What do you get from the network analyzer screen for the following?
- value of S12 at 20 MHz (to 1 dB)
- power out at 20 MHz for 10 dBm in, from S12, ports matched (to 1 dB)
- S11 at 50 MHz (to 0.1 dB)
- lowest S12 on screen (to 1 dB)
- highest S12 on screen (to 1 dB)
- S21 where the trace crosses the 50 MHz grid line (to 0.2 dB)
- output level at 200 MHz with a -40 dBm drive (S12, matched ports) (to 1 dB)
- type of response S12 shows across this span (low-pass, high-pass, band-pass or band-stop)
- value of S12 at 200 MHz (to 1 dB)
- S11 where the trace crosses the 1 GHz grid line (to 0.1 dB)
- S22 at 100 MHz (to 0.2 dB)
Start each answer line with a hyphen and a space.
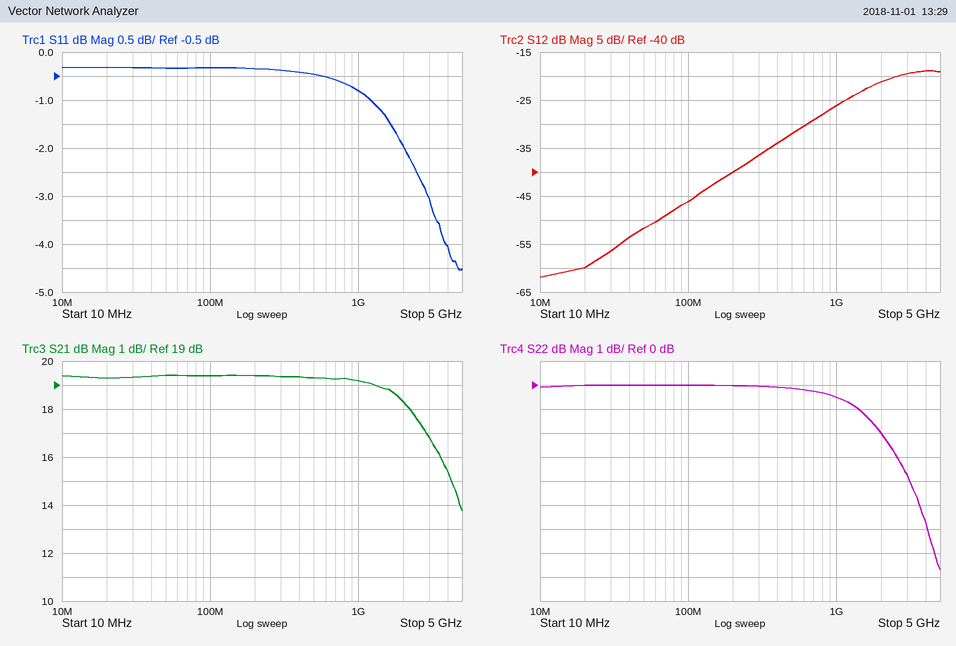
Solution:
- -60 dB
- -50 dBm
- -0.3 dB
- -62 dB
- -19 dB
- 19.4 dB
- -80 dBm
- high-pass
- -40 dB
- -0.8 dB
- 0.0 dB
